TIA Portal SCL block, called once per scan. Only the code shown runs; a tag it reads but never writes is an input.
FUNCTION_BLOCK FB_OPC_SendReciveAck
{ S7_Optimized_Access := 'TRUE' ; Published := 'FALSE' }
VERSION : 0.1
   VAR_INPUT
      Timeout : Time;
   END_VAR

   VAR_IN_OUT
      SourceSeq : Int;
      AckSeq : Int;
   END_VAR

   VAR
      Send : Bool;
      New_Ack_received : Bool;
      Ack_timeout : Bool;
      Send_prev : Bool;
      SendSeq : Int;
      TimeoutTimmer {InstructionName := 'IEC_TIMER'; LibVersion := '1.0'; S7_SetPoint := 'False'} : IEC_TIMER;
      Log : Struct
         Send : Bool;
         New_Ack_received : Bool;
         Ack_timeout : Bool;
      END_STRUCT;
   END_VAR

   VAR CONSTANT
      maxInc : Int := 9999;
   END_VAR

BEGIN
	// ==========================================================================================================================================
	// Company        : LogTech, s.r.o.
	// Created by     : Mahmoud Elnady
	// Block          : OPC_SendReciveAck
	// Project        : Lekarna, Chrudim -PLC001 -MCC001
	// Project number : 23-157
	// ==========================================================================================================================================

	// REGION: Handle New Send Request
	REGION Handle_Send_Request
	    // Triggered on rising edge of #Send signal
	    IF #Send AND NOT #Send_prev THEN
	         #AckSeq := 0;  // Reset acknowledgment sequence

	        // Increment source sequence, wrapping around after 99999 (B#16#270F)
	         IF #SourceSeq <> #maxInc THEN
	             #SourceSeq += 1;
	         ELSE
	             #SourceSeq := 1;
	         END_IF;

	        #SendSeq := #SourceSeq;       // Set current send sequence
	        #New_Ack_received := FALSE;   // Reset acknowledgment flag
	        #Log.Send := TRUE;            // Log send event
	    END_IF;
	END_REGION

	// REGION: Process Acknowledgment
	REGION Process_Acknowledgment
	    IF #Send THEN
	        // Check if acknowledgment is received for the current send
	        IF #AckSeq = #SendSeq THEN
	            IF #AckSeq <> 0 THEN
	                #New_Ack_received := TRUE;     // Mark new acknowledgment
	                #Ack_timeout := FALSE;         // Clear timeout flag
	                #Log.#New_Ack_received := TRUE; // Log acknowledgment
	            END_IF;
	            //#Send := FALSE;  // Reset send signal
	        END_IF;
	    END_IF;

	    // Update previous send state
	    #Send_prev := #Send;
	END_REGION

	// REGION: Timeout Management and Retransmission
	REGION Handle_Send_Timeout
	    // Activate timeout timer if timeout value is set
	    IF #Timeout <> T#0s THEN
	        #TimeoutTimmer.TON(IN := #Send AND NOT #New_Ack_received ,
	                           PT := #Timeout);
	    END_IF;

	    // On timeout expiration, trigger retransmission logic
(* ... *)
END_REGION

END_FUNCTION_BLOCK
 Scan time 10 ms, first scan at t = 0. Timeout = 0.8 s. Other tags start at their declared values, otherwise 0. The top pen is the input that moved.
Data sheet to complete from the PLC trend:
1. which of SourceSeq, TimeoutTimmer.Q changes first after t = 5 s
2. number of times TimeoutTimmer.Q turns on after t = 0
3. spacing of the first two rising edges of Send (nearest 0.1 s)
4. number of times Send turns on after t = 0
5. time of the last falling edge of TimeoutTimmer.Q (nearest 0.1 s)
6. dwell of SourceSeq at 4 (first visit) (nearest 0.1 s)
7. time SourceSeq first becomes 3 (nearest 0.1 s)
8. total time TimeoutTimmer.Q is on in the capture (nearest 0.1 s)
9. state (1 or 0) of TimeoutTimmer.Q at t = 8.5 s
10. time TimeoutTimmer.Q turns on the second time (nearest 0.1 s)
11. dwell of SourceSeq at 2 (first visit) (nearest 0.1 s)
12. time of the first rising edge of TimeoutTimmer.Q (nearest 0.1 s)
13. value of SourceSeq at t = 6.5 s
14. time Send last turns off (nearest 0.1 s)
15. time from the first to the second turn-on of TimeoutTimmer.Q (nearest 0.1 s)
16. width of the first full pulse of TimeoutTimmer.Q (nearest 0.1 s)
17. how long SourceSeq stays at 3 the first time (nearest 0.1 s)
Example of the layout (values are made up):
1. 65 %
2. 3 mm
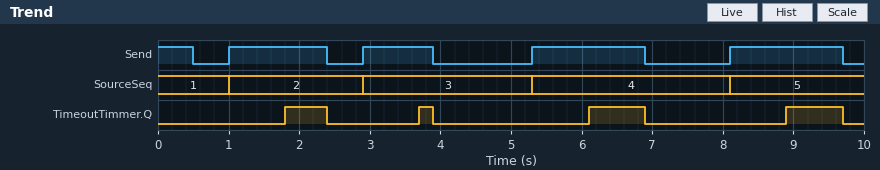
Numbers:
1. SourceSeq
2. 4
3. 1.9 s
4. 4
5. 9.7 s
6. 2.8 s
7. 2.9 s
8. 2.4 s
9. 0
10. 3.7 s
11. 1.9 s
12. 1.8 s
13. 4
14. 9.7 s
15. 1.9 s
16. 0.6 s
17. 2.4 s
